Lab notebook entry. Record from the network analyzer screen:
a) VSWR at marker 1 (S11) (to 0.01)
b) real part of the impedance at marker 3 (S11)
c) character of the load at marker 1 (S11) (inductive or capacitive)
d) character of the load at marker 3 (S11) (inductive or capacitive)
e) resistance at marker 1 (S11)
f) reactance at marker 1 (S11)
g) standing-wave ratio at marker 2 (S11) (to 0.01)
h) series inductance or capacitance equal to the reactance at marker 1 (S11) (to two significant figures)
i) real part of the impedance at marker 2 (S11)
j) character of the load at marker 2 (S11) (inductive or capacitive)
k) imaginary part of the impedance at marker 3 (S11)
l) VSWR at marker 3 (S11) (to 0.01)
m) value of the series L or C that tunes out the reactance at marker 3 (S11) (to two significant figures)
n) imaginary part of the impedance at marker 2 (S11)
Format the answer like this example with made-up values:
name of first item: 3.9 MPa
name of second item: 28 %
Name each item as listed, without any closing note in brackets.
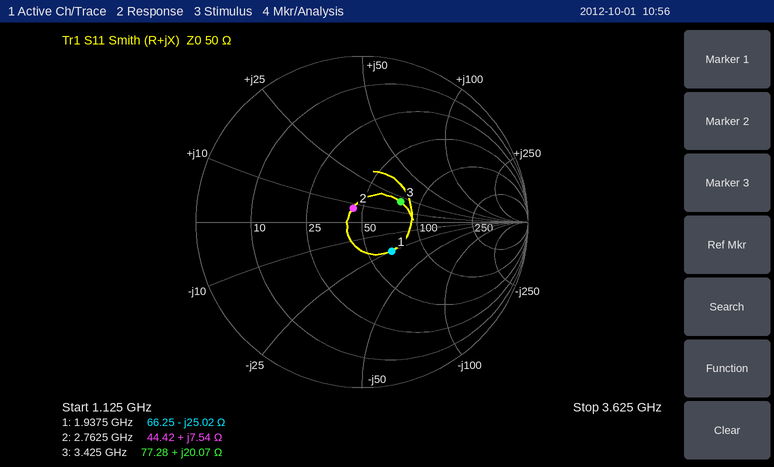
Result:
VSWR at marker 1 (S11): 1.67
real part of the impedance at marker 3: 77.28 Ω
character of the load at marker 1 (S11): capacitive
character of the load at marker 3 (S11): inductive
resistance at marker 1: 66.25 Ω
reactance at marker 1: -25.02 Ω
standing-wave ratio at marker 2 (S11): 1.22
series inductance or capacitance equal to the reactance at marker 1 (S11): 3.3 pF
real part of the impedance at marker 2: 44.42 Ω
character of the load at marker 2 (S11): inductive
imaginary part of the impedance at marker 3: +20.07 Ω
VSWR at marker 3 (S11): 1.71
value of the series L or C that tunes out the reactance at marker 3 (S11): 2.3 pF
imaginary part of the impedance at marker 2: +7.54 Ω
